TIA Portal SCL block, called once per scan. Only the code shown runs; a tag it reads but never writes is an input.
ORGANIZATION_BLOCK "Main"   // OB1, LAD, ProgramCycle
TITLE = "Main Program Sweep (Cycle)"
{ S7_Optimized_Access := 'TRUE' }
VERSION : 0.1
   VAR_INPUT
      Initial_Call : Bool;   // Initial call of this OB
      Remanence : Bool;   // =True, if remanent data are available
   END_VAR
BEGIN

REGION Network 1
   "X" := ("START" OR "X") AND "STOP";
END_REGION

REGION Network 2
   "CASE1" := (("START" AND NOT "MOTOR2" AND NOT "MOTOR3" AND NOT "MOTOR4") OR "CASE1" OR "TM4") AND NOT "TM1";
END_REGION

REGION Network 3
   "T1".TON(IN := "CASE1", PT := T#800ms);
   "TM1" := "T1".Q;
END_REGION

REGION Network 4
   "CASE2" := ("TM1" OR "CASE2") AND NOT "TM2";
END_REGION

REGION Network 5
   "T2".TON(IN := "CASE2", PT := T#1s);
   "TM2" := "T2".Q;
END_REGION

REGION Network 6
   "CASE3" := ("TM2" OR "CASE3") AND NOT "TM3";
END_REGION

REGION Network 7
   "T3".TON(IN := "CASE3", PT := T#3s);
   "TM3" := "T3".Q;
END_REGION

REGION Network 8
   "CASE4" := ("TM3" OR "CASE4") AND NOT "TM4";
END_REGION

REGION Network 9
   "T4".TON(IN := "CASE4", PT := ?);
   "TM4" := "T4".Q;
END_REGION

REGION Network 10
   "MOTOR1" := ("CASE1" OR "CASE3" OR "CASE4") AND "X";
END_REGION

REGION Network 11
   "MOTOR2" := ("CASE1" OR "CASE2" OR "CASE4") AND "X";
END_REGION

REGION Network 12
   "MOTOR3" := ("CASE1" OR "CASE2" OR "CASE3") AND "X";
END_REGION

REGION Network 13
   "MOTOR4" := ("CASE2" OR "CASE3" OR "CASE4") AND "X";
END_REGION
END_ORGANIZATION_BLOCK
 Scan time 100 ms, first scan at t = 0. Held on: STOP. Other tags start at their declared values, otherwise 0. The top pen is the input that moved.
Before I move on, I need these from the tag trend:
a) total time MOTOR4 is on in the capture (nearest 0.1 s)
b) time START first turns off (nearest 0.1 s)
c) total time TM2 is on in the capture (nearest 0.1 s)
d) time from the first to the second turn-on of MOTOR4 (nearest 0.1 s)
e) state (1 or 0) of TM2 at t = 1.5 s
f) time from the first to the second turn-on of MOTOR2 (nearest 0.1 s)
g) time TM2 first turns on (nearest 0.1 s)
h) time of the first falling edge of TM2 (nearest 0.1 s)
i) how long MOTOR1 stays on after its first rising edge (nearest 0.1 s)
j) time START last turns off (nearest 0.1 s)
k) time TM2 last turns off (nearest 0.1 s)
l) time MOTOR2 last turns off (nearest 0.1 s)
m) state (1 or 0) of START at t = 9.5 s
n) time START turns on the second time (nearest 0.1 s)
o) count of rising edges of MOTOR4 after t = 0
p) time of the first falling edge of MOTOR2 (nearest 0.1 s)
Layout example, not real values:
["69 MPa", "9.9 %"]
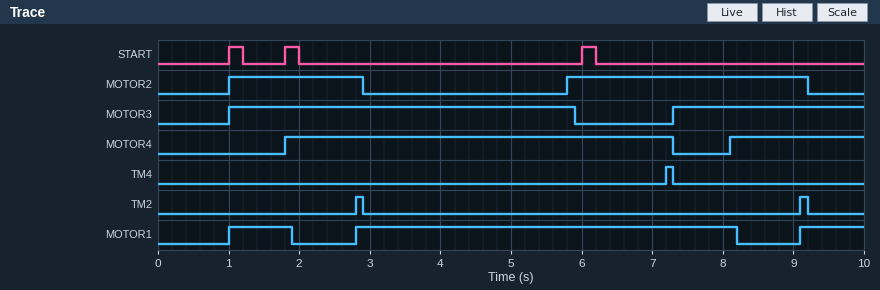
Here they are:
["7.4 s", "1.2 s", "0.2 s", "6.3 s", "0", "4.8 s", "2.8 s", "2.9 s", "0.9 s", "6.2 s", "9.2 s", "9.2 s", "0", "1.8 s", "2", "2.9 s"]
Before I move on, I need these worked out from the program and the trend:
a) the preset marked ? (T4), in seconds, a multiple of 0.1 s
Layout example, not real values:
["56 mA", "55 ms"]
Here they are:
["1.4 s"]
